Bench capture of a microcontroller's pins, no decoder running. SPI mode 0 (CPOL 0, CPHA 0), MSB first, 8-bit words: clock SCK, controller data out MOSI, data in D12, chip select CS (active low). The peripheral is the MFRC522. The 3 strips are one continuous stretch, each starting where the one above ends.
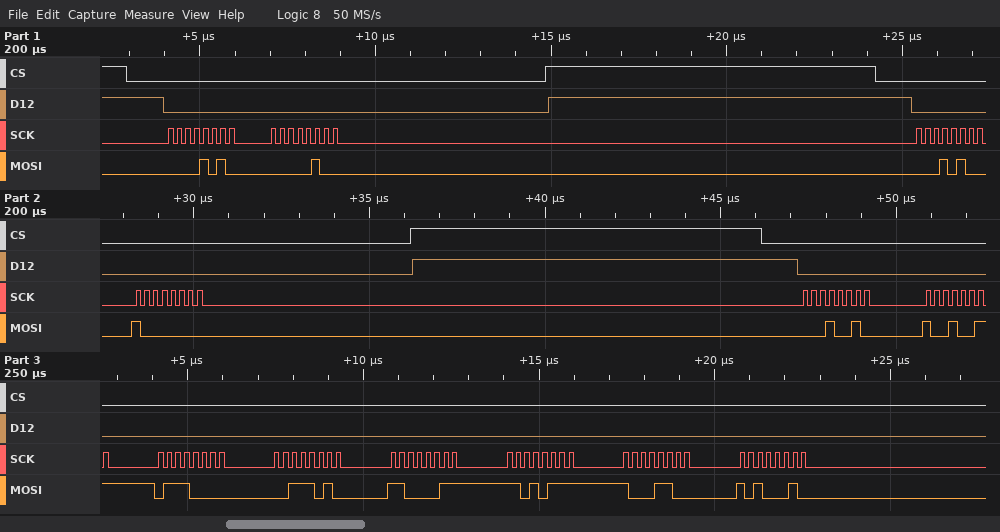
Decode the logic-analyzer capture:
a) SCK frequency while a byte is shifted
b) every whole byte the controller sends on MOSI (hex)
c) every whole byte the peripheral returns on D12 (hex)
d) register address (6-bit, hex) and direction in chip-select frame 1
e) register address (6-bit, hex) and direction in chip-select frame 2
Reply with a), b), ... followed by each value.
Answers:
a) 4 MHz
b) 0x0A 0x04 0x14 0x80 0x12 0x93 0x70 0x3A 0xC3 0xD7 0x8C 0xA2
c) 0x00 0x00 0x00 0x00 0x00 0x00 0x00 0x00 0x00 0x00 0x00 0x00
d) 0x05 write
e) 0x0A write
